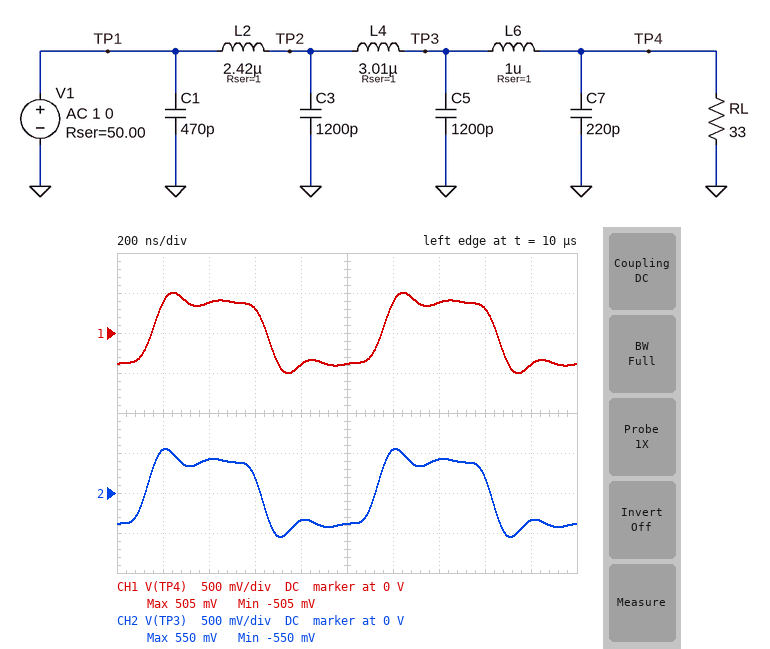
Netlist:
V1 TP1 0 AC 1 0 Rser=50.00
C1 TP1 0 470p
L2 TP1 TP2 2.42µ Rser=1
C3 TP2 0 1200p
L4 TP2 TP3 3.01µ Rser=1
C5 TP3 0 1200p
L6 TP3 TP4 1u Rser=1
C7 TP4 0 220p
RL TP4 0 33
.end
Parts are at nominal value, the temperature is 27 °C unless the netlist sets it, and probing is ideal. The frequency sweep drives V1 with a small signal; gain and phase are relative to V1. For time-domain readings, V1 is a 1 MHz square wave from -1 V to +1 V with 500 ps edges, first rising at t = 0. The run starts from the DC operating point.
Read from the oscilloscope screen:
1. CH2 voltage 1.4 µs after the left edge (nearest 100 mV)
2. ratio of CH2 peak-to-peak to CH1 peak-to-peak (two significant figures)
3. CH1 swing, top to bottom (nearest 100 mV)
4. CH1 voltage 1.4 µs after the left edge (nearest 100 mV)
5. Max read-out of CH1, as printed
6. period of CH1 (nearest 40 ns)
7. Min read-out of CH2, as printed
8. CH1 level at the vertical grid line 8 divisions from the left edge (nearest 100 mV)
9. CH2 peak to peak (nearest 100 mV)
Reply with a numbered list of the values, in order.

1. 400 mV
2. 1.1
3. 1.0 V
4. 400 mV
5. 505 mV
6. 1.00 µs
7. -550 mV
8. 300 mV
9. 1.1 V
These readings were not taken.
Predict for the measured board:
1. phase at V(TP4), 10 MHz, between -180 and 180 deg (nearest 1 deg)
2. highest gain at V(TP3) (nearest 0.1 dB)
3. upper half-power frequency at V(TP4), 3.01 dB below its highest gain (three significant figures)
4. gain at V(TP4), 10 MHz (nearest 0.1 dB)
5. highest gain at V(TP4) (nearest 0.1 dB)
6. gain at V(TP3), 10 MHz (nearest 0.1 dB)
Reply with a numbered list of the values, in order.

1. -124 deg
2. -7.2 dB
3. 5.01 MHz
4. -49.3 dB
5. -8.3 dB
6. -43.6 dB
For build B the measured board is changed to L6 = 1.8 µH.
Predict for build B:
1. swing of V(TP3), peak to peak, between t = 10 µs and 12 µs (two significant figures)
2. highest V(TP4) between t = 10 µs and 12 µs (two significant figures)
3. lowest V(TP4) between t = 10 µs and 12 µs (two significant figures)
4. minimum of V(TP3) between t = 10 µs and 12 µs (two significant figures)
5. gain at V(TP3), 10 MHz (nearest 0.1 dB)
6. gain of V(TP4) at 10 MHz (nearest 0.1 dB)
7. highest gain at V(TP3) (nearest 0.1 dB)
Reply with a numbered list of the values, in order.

1. 1.4 V
2. 530 mV
3. -530 mV
4. -700 mV
5. -44.4 dB
6. -55.2 dB
7. -3.8 dB
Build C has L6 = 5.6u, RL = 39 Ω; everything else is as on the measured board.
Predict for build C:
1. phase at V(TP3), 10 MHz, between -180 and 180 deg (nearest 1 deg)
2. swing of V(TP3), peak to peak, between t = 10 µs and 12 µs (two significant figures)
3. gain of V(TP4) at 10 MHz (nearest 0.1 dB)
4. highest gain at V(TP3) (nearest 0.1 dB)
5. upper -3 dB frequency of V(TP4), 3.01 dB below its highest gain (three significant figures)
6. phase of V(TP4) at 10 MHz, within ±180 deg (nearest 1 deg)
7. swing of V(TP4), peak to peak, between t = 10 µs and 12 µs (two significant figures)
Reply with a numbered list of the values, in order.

1. -47 deg
2. 2.1 V
3. -65.1 dB
4. -0.3 dB
5. 3.31 MHz
6. -160 deg
7. 960 mV
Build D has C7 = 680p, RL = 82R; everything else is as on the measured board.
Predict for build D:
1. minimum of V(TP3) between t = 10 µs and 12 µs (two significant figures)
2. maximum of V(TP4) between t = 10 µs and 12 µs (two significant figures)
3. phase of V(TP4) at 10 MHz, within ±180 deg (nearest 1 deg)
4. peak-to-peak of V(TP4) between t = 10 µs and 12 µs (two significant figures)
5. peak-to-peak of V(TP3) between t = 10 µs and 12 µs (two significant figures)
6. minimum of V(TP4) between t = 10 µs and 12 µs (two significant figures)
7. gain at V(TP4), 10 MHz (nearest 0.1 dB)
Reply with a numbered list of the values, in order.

1. -640 mV
2. 690 mV
3. 164 deg
4. 1.4 V
5. 1.3 V
6. -690 mV
7. -47.4 dB
